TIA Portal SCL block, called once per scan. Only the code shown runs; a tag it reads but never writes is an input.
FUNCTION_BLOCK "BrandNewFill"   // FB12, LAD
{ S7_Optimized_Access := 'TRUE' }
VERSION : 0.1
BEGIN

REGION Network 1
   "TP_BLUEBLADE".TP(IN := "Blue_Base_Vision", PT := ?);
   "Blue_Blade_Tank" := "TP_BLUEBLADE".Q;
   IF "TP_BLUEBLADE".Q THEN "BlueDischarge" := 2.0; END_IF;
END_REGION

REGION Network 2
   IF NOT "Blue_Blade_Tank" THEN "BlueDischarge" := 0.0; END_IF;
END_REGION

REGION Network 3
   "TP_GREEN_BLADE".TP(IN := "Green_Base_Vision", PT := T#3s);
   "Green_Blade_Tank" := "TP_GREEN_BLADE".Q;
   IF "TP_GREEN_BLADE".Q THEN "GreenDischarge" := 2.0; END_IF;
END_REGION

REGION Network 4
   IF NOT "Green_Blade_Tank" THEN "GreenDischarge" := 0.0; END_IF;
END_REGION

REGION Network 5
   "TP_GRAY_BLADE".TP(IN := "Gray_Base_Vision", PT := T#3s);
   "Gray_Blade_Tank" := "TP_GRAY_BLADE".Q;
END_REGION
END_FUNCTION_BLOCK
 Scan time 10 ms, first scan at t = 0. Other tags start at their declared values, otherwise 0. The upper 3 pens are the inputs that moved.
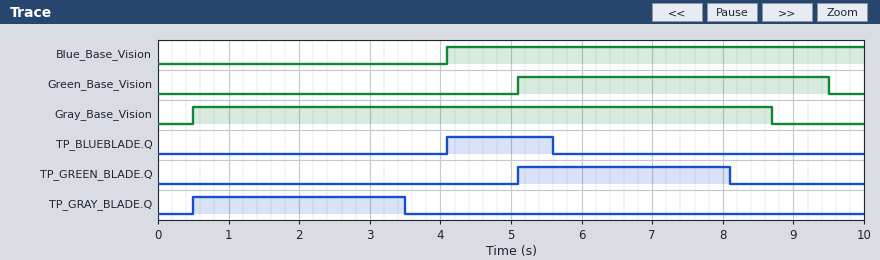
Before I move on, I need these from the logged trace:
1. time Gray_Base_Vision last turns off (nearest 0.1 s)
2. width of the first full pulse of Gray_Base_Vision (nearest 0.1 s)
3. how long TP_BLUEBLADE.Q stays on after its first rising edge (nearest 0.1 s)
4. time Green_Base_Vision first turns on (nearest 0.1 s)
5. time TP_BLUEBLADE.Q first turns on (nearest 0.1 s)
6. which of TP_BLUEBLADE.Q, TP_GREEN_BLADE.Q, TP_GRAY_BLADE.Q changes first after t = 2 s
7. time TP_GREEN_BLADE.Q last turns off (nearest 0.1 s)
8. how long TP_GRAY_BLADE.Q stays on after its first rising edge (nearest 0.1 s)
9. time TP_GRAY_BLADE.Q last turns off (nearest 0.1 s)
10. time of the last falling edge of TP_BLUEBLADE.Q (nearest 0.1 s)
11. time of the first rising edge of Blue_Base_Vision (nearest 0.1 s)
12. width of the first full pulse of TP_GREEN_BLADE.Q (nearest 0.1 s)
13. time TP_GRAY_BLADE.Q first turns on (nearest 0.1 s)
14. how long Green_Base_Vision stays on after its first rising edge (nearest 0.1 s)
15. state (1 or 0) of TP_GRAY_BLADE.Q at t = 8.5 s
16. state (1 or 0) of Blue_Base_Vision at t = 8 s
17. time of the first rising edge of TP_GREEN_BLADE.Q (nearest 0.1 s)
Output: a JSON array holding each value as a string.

["8.7 s", "8.2 s", "1.5 s", "5.1 s", "4.1 s", "TP_GRAY_BLADE.Q", "8.1 s", "3.0 s", "3.5 s", "5.6 s", "4.1 s", "3.0 s", "0.5 s", "4.4 s", "0", "1", "5.1 s"]
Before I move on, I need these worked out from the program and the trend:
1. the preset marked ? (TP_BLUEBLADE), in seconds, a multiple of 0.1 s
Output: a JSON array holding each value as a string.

["1.5 s"]
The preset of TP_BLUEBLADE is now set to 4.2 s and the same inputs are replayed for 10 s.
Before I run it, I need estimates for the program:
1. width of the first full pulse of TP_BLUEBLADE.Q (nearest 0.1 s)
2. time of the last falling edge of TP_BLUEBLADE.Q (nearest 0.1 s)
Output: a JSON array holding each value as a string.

["4.2 s", "8.3 s"]
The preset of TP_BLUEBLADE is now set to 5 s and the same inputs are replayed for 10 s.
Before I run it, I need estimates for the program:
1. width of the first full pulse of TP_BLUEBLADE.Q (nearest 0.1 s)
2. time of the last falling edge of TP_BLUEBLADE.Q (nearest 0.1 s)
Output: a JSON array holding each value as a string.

["5.0 s", "9.1 s"]
